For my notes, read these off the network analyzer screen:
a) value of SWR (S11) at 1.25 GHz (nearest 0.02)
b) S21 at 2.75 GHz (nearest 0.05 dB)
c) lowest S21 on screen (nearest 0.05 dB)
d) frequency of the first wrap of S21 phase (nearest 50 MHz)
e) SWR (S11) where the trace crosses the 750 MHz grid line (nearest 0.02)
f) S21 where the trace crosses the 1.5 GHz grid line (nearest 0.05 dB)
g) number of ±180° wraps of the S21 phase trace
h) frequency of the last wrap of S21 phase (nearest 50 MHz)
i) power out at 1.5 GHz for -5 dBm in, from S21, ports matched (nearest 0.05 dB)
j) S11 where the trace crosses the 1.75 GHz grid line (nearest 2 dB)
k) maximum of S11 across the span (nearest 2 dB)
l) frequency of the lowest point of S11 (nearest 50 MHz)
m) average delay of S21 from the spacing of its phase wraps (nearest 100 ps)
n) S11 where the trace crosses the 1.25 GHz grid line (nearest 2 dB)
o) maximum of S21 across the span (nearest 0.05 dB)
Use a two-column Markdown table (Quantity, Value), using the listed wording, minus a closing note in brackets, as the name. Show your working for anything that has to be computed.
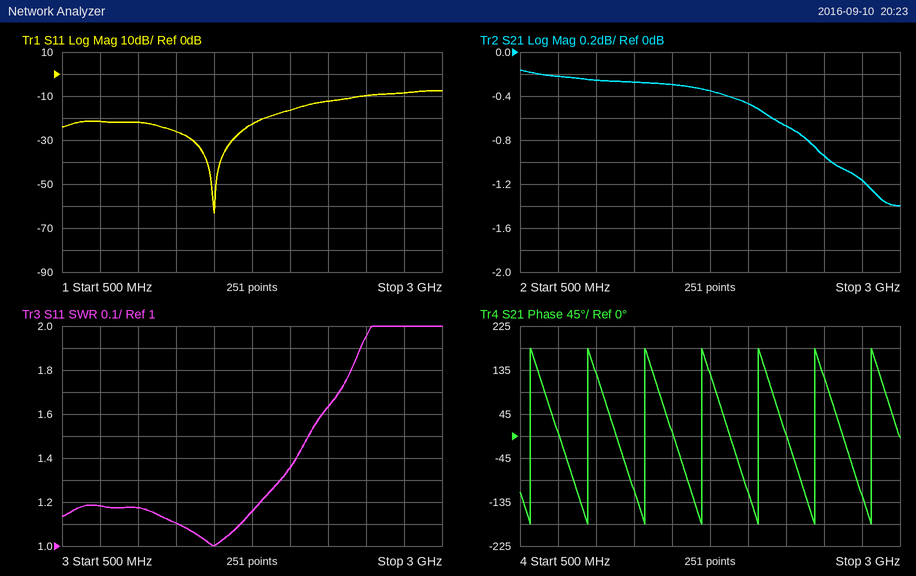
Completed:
| Quantity | Value |
|---|---|
| value of SWR (S11) at 1.25 GHz | 1.10 |
| S21 at 2.75 GHz | -1.15 dB |
| lowest S21 on screen | -1.40 dB |
| frequency of the first wrap of S21 phase | 550 MHz |
| SWR (S11) where the trace crosses the 750 MHz grid line | 1.18 |
| S21 where the trace crosses the 1.5 GHz grid line | -0.30 dB |
| number of ±180° wraps of the S21 phase trace | 7 |
| frequency of the last wrap of S21 phase | 2.80 GHz |
| power out at 1.5 GHz for -5 dBm in, from S21, ports matched | -5 dBm + (-0.30 dB) = -5.30 dBm |
| S11 where the trace crosses the 1.75 GHz grid line | -22 dB |
| maximum of S11 across the span | -8 dB |
| frequency of the lowest point of S11 | 1.50 GHz |
| average delay of S21 from the spacing of its phase wraps | 6 cycles / (2.80 GHz − 550 MHz) ≈ 2.7 ns |
| S11 where the trace crosses the 1.25 GHz grid line | -26 dB |
| maximum of S21 across the span | -0.15 dB |
